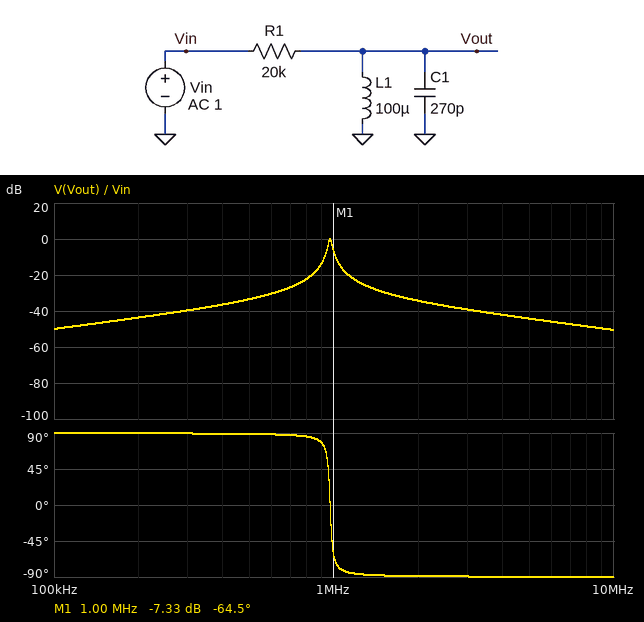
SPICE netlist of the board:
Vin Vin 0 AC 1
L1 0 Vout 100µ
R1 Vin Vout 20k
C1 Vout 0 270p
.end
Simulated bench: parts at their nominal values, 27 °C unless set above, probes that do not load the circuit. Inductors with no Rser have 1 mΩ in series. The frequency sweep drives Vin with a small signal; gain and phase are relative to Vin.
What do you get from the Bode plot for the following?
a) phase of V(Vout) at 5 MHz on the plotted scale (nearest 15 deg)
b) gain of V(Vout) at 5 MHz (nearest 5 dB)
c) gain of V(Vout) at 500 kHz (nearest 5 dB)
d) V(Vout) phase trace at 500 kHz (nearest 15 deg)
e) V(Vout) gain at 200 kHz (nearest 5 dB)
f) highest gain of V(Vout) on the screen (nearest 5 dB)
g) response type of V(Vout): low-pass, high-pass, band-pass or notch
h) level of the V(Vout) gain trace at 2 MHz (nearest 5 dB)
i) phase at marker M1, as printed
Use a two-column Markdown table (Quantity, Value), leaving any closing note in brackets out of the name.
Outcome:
| Quantity | Value |
|---|---|
| phase of V(Vout) at 5 MHz on the plotted scale | -90 deg |
| gain of V(Vout) at 5 MHz | -45 dB |
| gain of V(Vout) at 500 kHz | -35 dB |
| V(Vout) phase trace at 500 kHz | 90 deg |
| V(Vout) gain at 200 kHz | -45 dB |
| highest gain of V(Vout) on the screen | 0 dB |
| response type of V(Vout): low-pass, high-pass, band-pass or notch | band-pass |
| level of the V(Vout) gain trace at 2 MHz | -35 dB |
| phase at marker M1, as printed | -64.5 deg |
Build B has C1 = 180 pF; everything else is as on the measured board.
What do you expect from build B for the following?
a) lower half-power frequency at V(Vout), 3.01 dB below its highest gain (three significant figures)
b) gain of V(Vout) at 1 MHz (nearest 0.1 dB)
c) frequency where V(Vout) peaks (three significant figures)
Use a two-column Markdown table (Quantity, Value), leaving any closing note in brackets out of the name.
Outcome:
| Quantity | Value |
|---|---|
| lower half-power frequency at V(Vout), 3.01 dB below its highest gain | 1.16 MHz |
| gain of V(Vout) at 1 MHz | -19.3 dB |
| frequency where V(Vout) peaks | 1.19 MHz |
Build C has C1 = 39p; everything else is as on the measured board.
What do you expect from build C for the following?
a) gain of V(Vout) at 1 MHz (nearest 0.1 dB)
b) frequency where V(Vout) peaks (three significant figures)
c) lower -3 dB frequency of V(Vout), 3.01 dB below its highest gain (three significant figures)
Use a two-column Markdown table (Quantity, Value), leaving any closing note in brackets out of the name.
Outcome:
| Quantity | Value |
|---|---|
| gain of V(Vout) at 1 MHz | -28.6 dB |
| frequency where V(Vout) peaks | 2.55 MHz |
| lower -3 dB frequency of V(Vout), 3.01 dB below its highest gain | 2.45 MHz |
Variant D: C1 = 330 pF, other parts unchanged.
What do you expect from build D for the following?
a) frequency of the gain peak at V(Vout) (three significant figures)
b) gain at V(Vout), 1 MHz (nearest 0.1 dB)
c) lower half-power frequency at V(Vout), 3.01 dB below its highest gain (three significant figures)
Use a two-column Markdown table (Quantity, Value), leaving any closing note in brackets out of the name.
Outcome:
| Quantity | Value |
|---|---|
| frequency of the gain peak at V(Vout) | 876 kHz |
| gain at V(Vout), 1 MHz | -19.7 dB |
| lower half-power frequency at V(Vout), 3.01 dB below its highest gain | 864 kHz |
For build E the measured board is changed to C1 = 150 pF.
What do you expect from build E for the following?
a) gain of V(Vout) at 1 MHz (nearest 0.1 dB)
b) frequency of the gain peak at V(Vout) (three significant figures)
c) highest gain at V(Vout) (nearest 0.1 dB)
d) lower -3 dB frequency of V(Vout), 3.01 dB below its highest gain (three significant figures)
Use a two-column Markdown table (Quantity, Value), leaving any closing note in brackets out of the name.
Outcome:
| Quantity | Value |
|---|---|
| gain of V(Vout) at 1 MHz | -22.3 dB |
| frequency of the gain peak at V(Vout) | 1.30 MHz |
| highest gain at V(Vout) | 0 dB |
| lower -3 dB frequency of V(Vout), 3.01 dB below its highest gain | 1.27 MHz |
